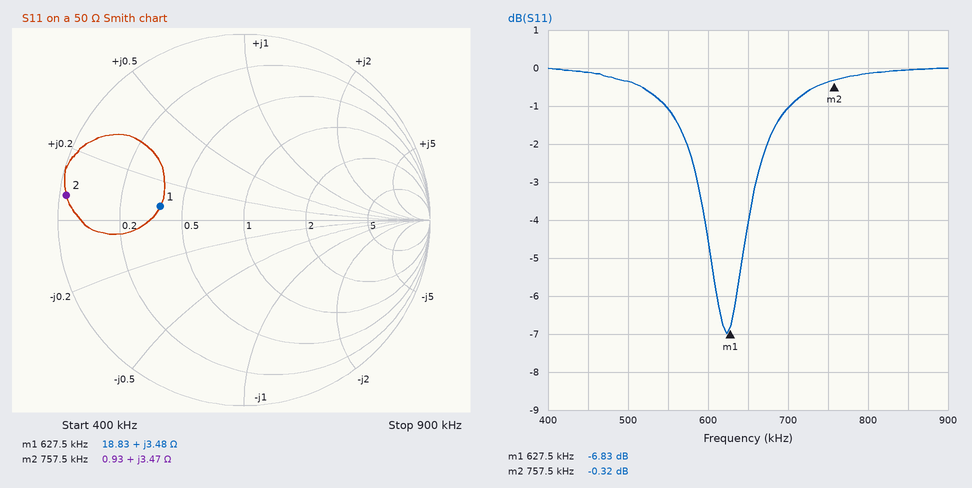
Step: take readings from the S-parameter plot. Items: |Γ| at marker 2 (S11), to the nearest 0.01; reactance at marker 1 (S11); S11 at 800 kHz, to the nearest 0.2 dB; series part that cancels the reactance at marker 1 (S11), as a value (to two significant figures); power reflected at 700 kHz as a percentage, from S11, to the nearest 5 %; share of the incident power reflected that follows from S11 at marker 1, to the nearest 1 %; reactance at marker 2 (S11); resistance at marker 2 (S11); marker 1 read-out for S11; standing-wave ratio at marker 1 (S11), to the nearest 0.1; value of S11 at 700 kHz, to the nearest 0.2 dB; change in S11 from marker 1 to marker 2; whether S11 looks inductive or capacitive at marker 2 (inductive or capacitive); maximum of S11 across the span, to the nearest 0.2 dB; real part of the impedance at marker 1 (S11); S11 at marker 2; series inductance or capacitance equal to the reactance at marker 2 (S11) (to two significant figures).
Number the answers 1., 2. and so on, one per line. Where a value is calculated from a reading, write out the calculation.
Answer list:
1. 0.96
2. +3.48 Ω
3. -0.2 dB
4. C = 1/(2π × 627.5 kHz × 3.48 Ω) ≈ 73 nF
5. 10^(-1/10) ≈ 79.4 %, so 80 % to the nearest 5 %
6. 10^(-6.83/10) ≈ 21 %
7. +3.47 Ω
8. 0.93 Ω
9. -6.83 dB
10. 2.7
11. -1.0 dB
12. -0.32 − (-6.83) = 6.51 dB
13. inductive
14. 0.0 dB
15. 18.83 Ω
16. -0.32 dB
17. L = 3.47 Ω/(2π × 757.5 kHz) ≈ 729 nH, so 730 nH to two significant figures
